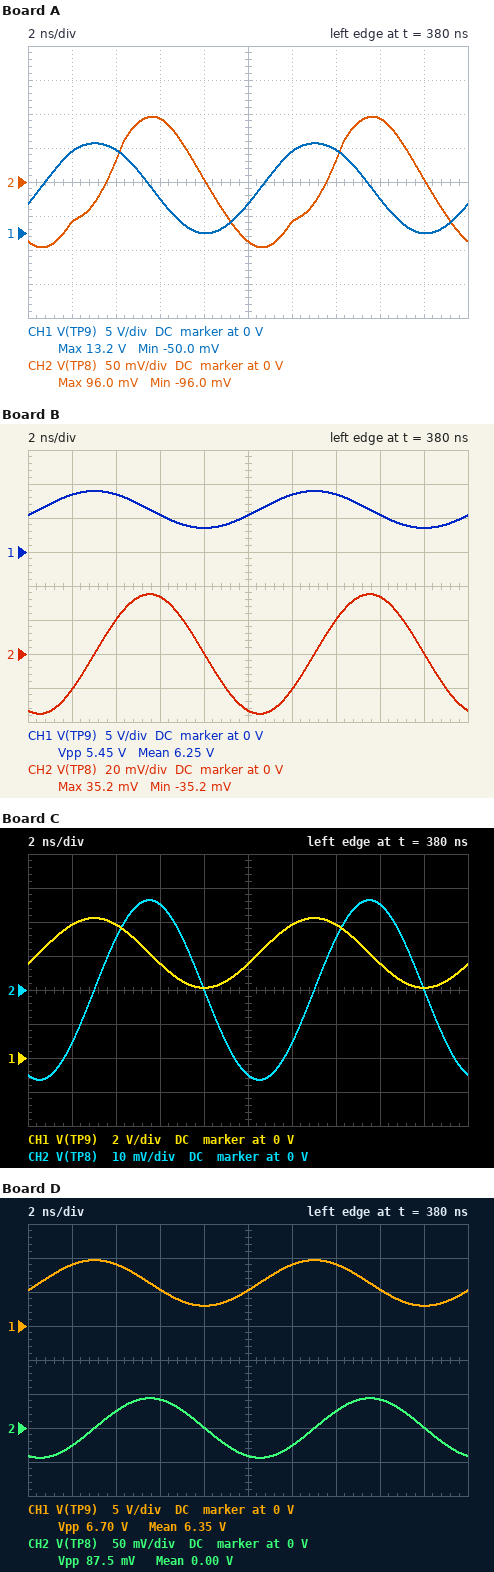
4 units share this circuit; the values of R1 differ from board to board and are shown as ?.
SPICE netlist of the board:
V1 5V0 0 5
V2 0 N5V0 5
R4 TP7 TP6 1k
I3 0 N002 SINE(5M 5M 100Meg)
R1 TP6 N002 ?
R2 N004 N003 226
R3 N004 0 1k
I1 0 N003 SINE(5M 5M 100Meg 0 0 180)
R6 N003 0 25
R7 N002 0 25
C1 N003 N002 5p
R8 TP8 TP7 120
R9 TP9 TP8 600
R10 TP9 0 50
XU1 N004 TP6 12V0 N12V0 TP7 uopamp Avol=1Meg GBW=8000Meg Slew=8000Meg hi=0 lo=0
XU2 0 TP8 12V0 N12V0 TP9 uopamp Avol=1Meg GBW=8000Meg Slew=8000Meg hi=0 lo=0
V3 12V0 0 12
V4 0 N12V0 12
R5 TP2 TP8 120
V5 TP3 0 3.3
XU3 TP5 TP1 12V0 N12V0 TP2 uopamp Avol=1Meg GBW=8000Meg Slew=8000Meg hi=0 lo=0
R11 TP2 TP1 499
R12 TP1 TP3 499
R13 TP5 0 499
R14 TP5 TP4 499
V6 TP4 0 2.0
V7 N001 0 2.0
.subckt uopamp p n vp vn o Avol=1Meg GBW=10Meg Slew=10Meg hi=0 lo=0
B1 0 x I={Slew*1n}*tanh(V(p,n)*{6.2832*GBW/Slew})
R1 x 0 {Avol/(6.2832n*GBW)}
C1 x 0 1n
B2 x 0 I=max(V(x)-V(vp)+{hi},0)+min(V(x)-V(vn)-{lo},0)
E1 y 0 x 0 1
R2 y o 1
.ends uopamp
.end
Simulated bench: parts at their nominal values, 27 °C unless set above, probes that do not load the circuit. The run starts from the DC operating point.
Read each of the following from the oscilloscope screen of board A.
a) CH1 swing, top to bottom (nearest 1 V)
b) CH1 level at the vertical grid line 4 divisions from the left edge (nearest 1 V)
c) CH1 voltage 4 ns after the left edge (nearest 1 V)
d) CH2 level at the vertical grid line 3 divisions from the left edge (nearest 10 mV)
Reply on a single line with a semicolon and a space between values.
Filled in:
13 V; 0 V; 12 V; 90 mV
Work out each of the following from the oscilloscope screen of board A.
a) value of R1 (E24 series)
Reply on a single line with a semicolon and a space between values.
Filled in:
150 Ω
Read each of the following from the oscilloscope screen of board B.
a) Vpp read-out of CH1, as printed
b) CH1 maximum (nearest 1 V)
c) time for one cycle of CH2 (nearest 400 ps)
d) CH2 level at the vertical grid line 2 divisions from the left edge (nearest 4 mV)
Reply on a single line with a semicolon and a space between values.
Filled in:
5.45 V; 9 V; 10.0 ns; 20 mV
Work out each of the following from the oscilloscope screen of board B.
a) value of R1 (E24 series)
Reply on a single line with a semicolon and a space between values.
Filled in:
470 Ω
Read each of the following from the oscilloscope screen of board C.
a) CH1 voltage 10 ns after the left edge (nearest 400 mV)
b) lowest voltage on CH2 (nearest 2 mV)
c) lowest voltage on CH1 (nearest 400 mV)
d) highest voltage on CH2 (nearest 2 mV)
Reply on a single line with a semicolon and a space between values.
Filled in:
5.6 V; -26 mV; 4.0 V; 26 mV
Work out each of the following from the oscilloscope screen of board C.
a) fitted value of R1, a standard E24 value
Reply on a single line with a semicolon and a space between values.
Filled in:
680 Ω
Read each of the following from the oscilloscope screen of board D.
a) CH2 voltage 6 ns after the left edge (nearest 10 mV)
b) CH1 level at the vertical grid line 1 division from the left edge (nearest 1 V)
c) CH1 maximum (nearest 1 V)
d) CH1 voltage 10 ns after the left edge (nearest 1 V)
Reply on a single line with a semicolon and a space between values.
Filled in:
40 mV; 9 V; 10 V; 5 V
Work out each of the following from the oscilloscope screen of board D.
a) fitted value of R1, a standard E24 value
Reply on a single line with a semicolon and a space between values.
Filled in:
360 Ω
